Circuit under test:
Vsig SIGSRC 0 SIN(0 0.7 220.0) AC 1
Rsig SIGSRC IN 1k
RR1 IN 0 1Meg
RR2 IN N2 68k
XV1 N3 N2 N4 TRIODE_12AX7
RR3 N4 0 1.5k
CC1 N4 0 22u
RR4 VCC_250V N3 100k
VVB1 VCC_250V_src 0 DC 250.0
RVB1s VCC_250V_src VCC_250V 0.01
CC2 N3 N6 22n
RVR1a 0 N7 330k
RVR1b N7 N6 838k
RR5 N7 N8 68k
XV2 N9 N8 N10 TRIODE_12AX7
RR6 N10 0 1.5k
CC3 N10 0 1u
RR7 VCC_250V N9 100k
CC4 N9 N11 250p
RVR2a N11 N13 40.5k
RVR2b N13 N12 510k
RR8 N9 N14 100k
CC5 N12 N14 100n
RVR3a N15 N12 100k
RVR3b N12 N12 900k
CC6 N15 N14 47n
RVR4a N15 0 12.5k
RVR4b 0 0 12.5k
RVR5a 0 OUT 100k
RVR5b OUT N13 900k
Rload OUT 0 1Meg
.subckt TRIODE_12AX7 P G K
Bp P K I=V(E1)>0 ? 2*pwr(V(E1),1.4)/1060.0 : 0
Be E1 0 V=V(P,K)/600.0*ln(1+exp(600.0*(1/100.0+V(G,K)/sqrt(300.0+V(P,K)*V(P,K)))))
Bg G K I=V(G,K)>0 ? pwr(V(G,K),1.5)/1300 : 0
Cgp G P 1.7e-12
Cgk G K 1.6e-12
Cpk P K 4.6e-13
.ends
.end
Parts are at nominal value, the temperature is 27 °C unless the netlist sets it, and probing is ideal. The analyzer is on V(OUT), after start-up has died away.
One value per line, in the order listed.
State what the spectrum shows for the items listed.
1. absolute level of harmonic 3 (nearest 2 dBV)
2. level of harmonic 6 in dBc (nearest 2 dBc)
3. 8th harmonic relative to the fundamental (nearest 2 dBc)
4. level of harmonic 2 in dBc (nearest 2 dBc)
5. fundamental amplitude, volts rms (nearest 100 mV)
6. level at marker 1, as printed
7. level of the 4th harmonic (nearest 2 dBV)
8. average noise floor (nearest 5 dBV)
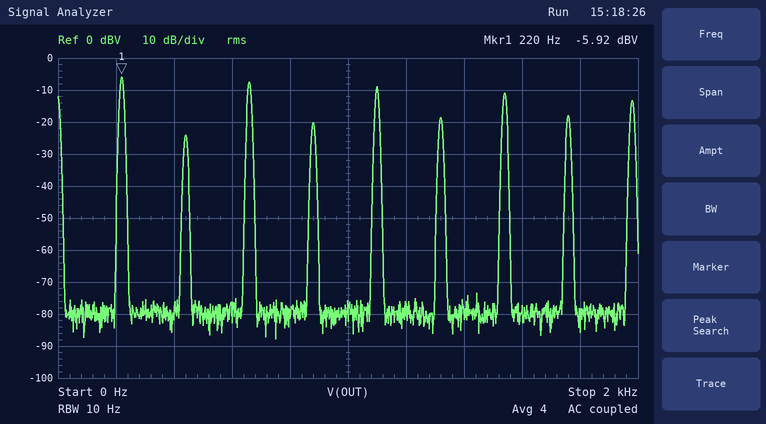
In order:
-8 dBV
-12 dBc
-12 dBc
-18 dBc
500 mV
-5.92 dBV
-20 dBV
-80 dBV
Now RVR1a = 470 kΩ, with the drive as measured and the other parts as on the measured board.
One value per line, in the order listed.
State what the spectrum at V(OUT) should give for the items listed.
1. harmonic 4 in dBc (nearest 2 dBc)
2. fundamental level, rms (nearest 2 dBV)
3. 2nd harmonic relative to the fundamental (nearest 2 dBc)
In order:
-12 dBc
-6 dBV
-16 dBc
